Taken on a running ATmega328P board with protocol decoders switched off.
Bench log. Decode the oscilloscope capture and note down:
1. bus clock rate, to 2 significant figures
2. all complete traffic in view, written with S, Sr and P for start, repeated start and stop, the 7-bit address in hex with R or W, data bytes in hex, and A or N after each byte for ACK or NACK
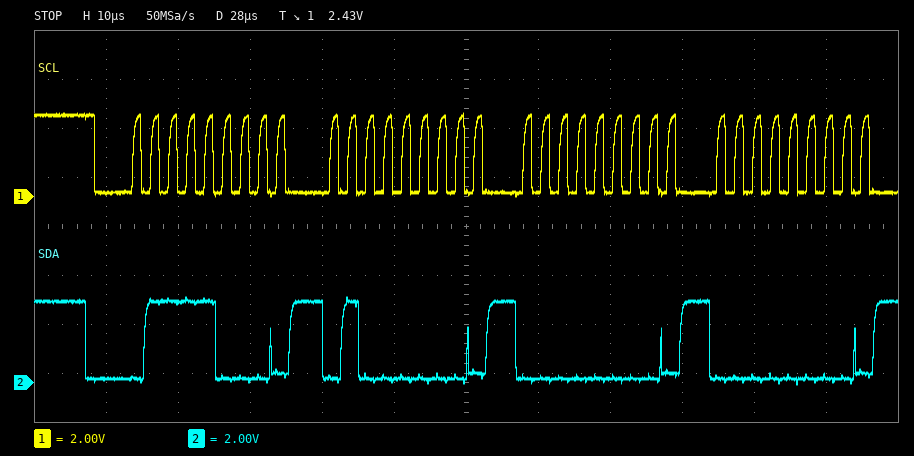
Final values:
400 kHz
S 3CW A 40 A 00 A 00 A
